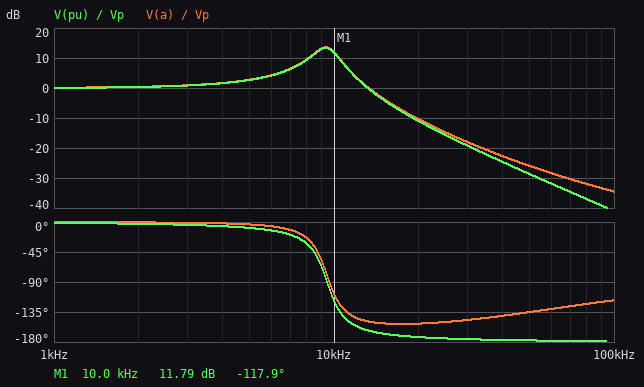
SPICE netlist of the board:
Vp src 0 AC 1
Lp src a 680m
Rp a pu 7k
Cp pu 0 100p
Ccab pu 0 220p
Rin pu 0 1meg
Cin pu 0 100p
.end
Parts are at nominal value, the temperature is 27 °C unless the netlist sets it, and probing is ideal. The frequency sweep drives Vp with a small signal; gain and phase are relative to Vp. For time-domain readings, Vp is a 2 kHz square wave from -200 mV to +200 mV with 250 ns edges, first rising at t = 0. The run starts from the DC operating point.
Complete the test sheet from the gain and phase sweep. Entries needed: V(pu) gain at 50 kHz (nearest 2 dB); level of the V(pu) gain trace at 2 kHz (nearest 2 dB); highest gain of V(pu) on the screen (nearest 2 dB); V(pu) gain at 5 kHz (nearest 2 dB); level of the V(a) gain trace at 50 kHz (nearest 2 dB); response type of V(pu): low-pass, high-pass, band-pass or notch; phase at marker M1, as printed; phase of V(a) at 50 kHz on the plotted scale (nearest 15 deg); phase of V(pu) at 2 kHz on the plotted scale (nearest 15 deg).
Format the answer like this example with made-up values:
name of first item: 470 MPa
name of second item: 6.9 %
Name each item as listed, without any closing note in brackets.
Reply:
V(pu) gain at 50 kHz: -28 dB
level of the V(pu) gain trace at 2 kHz: 0 dB
highest gain of V(pu) on the screen: 14 dB
V(pu) gain at 5 kHz: 2 dB
level of the V(a) gain trace at 50 kHz: -26 dB
response type of V(pu): low-pass, high-pass, band-pass or notch: low-pass
phase at marker M1, as printed: -117.9 deg
phase of V(a) at 50 kHz on the plotted scale: -135 deg
phase of V(pu) at 2 kHz on the plotted scale: 0 deg
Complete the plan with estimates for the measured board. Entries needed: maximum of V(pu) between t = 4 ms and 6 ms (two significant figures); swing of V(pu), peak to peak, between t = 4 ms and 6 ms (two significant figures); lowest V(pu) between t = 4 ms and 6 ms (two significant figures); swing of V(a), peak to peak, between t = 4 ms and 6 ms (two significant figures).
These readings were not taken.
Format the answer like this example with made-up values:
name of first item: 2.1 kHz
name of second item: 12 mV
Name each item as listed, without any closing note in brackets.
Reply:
maximum of V(pu) between t = 4 ms and 6 ms: 510 mV
swing of V(pu), peak to peak, between t = 4 ms and 6 ms: 1.0 V
lowest V(pu) between t = 4 ms and 6 ms: -510 mV
swing of V(a), peak to peak, between t = 4 ms and 6 ms: 1.0 V
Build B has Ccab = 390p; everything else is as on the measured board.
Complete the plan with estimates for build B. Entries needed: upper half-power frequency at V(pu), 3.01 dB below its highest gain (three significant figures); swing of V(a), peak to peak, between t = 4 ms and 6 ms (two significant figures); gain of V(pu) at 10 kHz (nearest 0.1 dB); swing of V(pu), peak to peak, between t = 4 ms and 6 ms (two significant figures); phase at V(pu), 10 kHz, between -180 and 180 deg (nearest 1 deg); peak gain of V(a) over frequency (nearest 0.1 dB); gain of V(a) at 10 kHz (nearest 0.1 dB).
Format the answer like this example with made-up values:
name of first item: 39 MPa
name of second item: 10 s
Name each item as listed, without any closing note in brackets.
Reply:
upper half-power frequency at V(pu), 3.01 dB below its highest gain: 8.77 kHz
swing of V(a), peak to peak, between t = 4 ms and 6 ms: 860 mV
gain of V(pu) at 10 kHz: 3.7 dB
swing of V(pu), peak to peak, between t = 4 ms and 6 ms: 840 mV
phase at V(pu), 10 kHz, between -180 and 180 deg: -152 deg
peak gain of V(a) over frequency: 12.7 dB
gain of V(a) at 10 kHz: 4.1 dB
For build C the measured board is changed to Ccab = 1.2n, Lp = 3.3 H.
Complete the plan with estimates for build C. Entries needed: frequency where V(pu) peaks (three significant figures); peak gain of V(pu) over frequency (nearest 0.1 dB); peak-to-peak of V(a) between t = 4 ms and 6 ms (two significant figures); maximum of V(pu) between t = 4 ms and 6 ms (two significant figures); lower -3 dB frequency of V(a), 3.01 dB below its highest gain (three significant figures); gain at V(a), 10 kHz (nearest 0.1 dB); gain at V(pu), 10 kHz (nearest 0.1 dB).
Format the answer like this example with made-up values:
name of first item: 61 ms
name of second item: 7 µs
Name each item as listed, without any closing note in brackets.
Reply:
frequency where V(pu) peaks: 2.33 kHz
peak gain of V(pu) over frequency: 14.3 dB
peak-to-peak of V(a) between t = 4 ms and 6 ms: 1.6 V
maximum of V(pu) between t = 4 ms and 6 ms: 790 mV
lower -3 dB frequency of V(a), 3.01 dB below its highest gain: 2.09 kHz
gain at V(a), 10 kHz: -23.3 dB
gain at V(pu), 10 kHz: -24.7 dB
